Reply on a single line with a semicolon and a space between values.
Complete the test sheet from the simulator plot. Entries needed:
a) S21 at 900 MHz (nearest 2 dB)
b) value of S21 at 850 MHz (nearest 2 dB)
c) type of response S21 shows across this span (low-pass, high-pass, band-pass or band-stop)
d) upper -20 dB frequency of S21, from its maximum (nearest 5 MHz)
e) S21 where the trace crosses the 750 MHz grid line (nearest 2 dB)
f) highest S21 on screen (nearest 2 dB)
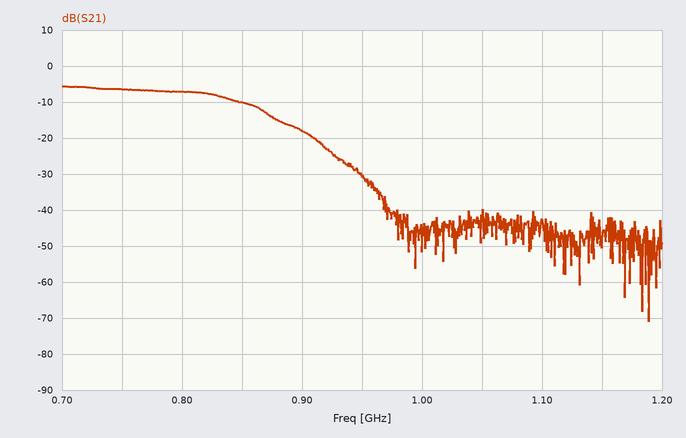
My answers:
-18 dB; -10 dB; low-pass; 930 MHz; -6 dB; -6 dB
